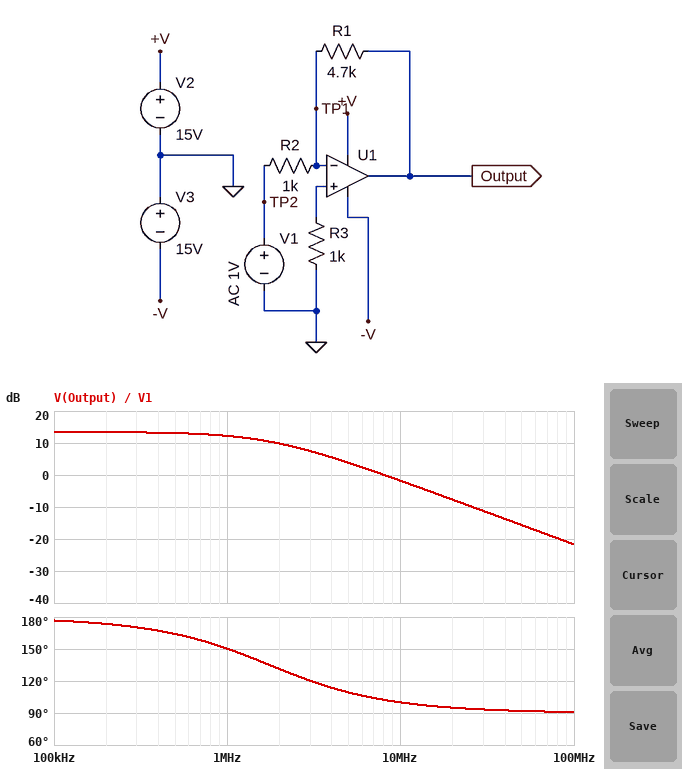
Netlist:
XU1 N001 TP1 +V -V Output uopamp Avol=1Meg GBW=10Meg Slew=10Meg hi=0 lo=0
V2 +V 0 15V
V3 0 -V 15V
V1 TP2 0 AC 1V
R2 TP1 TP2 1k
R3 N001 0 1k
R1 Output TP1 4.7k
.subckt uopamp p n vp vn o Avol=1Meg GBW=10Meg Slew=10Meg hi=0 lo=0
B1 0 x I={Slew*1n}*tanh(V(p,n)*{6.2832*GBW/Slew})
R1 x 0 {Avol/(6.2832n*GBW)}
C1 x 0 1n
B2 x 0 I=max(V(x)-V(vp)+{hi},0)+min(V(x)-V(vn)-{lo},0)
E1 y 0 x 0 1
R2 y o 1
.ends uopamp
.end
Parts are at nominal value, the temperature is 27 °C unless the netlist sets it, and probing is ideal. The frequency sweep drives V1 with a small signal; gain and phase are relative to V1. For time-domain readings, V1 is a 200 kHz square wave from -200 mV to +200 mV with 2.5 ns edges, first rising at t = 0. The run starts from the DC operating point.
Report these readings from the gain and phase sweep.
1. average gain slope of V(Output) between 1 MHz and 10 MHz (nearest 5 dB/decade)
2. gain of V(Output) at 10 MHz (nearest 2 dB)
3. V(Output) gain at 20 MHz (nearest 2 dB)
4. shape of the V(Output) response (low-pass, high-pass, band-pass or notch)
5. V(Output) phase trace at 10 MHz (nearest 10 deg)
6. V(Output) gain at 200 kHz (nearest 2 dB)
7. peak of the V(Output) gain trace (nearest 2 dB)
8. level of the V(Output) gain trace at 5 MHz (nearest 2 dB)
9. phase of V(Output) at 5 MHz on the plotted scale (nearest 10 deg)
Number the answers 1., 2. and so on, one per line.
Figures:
1. -15 dB/decade
2. -2 dB
3. -8 dB
4. low-pass
5. 100 deg
6. 14 dB
7. 14 dB
8. 4 dB
9. 110 deg
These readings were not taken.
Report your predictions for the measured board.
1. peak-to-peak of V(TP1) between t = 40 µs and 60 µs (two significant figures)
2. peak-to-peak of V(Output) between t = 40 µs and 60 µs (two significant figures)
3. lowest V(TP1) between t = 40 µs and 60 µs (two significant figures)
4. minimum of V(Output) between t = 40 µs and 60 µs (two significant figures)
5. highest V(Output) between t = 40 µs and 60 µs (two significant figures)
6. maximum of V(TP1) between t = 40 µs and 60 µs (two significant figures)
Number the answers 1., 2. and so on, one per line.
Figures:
1. 650 mV
2. 1.9 V
3. -330 mV
4. -940 mV
5. 940 mV
6. 330 mV
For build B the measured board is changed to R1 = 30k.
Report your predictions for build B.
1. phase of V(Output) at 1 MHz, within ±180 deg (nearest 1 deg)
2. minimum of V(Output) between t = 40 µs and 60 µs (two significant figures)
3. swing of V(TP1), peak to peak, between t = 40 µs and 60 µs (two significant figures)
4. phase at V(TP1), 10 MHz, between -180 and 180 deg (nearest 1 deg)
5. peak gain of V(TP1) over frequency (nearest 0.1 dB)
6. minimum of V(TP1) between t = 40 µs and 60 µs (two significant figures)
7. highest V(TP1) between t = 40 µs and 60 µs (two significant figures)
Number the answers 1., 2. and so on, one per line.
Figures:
1. 108 deg
2. -5.8 V
3. 760 mV
4. 2 deg
5. -0.3 dB
6. -380 mV
7. 380 mV
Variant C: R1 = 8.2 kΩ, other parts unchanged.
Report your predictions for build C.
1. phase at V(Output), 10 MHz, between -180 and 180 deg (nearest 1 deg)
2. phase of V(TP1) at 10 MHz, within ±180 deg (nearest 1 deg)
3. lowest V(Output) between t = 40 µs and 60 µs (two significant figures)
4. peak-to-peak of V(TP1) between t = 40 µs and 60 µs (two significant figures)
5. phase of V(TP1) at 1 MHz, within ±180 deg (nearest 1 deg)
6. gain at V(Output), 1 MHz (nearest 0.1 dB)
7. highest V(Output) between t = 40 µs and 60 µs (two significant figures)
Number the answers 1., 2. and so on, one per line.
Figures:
1. 96 deg
2. 6 deg
3. -1.6 V
4. 710 mV
5. 47 deg
6. 15.6 dB
7. 1.6 V
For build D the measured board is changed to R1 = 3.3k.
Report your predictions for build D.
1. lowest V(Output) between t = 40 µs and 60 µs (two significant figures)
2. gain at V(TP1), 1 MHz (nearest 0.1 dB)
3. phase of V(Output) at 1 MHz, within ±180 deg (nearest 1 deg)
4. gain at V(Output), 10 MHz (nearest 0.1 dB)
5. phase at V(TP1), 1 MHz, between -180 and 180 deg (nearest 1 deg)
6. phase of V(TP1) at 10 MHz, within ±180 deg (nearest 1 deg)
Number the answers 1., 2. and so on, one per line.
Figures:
1. -660 mV
2. -10.4 dB
3. 157 deg
4. -2.5 dB
5. 67 deg
6. 13 deg
